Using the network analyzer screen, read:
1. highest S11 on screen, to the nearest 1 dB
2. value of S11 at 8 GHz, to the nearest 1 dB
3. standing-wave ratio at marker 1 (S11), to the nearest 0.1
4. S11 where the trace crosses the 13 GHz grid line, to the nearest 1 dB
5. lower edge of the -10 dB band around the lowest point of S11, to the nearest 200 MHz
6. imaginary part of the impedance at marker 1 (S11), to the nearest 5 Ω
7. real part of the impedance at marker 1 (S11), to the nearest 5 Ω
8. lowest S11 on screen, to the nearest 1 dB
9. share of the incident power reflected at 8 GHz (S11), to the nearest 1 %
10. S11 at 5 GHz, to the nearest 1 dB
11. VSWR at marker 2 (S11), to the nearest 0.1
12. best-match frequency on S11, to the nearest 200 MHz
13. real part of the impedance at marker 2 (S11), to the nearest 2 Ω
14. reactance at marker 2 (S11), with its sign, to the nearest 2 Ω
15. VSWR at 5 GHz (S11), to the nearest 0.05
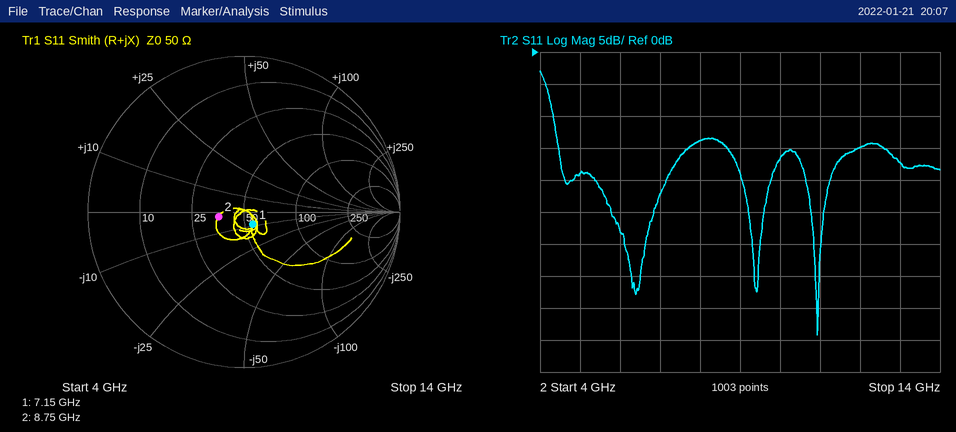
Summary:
-3 dB
-14 dB
1.2
-17 dB
4.4 GHz
-10 Ω
55 Ω
-44 dB
4 %
-19 dB
1.4
11.0 GHz
36 Ω
-2 Ω
1.25
